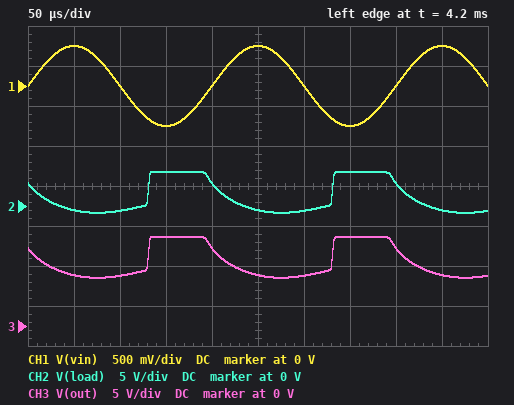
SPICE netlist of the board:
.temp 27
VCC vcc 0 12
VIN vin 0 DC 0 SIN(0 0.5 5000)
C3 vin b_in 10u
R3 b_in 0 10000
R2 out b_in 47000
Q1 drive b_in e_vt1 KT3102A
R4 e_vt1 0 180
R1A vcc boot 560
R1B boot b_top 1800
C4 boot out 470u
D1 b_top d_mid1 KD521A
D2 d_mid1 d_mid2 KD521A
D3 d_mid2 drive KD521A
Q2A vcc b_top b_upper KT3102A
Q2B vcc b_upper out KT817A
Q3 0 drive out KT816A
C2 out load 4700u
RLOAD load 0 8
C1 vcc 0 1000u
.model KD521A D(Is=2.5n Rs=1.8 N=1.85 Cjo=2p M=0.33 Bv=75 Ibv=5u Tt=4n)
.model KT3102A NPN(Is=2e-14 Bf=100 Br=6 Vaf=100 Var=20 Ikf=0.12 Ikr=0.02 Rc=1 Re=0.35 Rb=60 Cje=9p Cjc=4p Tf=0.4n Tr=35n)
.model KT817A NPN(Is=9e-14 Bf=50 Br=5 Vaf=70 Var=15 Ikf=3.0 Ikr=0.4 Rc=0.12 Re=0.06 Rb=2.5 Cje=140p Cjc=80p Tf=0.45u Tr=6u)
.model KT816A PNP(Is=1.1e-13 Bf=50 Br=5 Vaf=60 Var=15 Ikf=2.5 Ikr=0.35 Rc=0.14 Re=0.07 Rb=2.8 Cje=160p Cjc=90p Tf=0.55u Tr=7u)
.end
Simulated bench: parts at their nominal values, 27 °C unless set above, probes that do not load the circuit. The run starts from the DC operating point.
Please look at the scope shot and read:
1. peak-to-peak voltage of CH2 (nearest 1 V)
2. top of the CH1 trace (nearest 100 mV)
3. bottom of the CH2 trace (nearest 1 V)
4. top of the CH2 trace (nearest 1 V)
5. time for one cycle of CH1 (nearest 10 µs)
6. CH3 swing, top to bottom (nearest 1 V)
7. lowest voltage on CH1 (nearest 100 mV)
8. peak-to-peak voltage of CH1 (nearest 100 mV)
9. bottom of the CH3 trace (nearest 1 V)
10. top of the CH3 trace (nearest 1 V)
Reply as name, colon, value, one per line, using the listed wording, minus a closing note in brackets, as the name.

peak-to-peak voltage of CH2: 5 V
top of the CH1 trace: 500 mV
bottom of the CH2 trace: -1 V
top of the CH2 trace: 4 V
time for one cycle of CH1: 200 µs
CH3 swing, top to bottom: 5 V
lowest voltage on CH1: -500 mV
peak-to-peak voltage of CH1: 1.0 V
bottom of the CH3 trace: 6 V
top of the CH3 trace: 11 V
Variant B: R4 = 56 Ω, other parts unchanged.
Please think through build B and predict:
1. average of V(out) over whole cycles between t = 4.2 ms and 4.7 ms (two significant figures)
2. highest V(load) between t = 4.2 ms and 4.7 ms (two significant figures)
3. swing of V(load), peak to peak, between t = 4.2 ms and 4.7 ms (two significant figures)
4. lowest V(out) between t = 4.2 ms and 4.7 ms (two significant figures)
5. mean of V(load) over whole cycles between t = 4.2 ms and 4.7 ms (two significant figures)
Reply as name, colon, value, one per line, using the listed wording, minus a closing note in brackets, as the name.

average of V(out) over whole cycles between t = 4.2 ms and 4.7 ms: 7.2 V
highest V(load) between t = 4.2 ms and 4.7 ms: 5.2 V
swing of V(load), peak to peak, between t = 4.2 ms and 4.7 ms: 7.5 V
lowest V(out) between t = 4.2 ms and 4.7 ms: 3.6 V
mean of V(load) over whole cycles between t = 4.2 ms and 4.7 ms: 1.2 V
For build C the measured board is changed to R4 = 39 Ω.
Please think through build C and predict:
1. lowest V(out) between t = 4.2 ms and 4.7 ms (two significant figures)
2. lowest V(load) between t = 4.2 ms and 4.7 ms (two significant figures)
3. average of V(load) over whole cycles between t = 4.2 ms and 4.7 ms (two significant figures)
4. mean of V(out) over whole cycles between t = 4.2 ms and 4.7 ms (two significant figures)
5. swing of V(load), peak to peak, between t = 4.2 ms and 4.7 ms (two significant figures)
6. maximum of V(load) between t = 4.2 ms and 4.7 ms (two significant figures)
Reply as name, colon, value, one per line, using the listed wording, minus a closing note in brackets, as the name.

lowest V(out) between t = 4.2 ms and 4.7 ms: 2.6 V
lowest V(load) between t = 4.2 ms and 4.7 ms: -3.1 V
average of V(load) over whole cycles between t = 4.2 ms and 4.7 ms: 1.0 V
mean of V(out) over whole cycles between t = 4.2 ms and 4.7 ms: 6.7 V
swing of V(load), peak to peak, between t = 4.2 ms and 4.7 ms: 8.5 V
maximum of V(load) between t = 4.2 ms and 4.7 ms: 5.4 V
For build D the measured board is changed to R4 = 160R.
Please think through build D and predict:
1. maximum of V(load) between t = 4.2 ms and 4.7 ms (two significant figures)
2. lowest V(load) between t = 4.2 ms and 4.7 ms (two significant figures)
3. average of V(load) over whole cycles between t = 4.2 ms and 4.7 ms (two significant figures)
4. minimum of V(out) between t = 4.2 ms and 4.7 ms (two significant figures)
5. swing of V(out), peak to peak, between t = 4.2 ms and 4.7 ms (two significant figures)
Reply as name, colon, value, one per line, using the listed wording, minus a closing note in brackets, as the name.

maximum of V(load) between t = 4.2 ms and 4.7 ms: 4.4 V
lowest V(load) between t = 4.2 ms and 4.7 ms: -950 mV
average of V(load) over whole cycles between t = 4.2 ms and 4.7 ms: 1.4 V
minimum of V(out) between t = 4.2 ms and 4.7 ms: 5.8 V
swing of V(out), peak to peak, between t = 4.2 ms and 4.7 ms: 5.3 V
